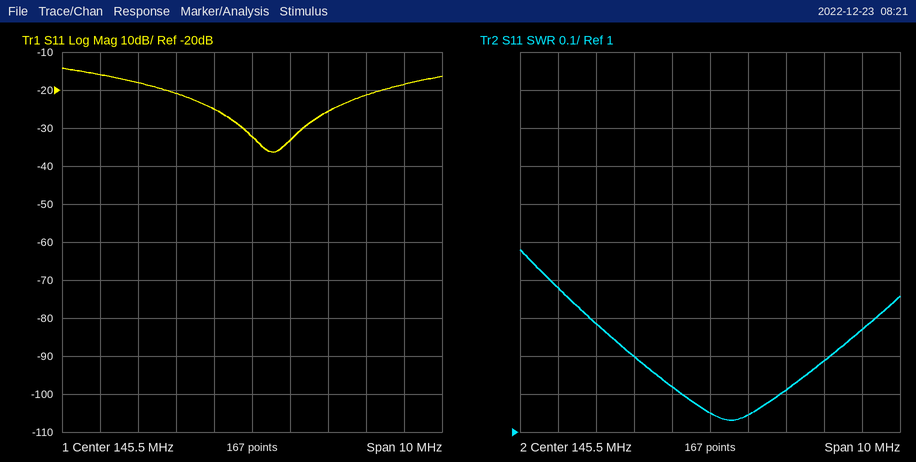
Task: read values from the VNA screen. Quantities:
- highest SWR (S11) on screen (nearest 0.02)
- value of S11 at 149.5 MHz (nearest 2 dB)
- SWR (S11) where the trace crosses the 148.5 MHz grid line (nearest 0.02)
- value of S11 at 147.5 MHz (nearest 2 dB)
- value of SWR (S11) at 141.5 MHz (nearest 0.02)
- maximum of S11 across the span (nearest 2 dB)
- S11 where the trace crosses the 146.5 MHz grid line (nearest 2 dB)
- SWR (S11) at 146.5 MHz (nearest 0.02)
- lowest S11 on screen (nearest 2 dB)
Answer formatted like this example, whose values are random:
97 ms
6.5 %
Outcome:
1.48
-18 dB
1.18
-26 dB
1.38
-14 dB
-34 dB
1.04
-36 dB
